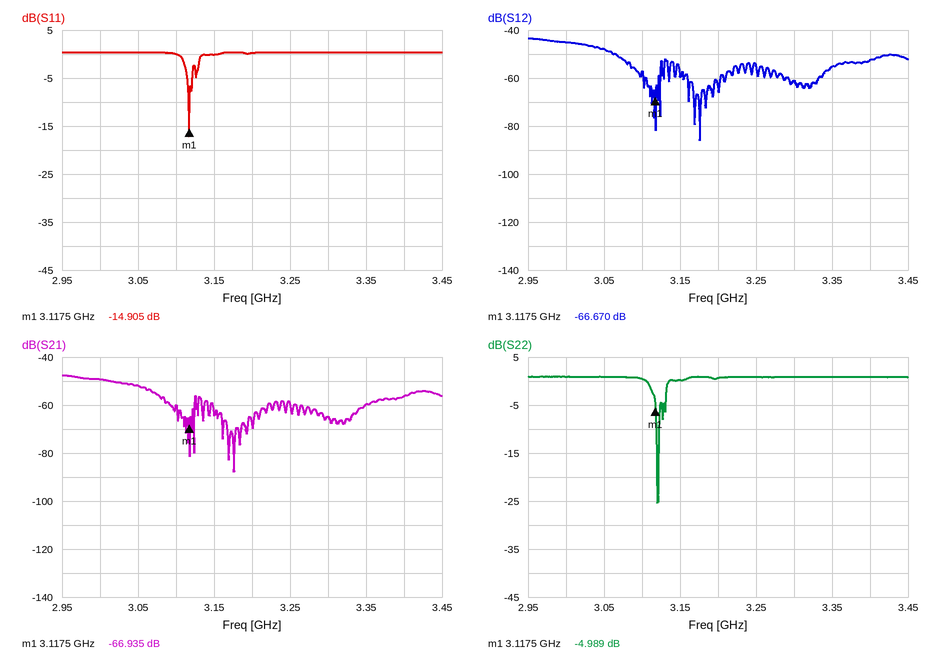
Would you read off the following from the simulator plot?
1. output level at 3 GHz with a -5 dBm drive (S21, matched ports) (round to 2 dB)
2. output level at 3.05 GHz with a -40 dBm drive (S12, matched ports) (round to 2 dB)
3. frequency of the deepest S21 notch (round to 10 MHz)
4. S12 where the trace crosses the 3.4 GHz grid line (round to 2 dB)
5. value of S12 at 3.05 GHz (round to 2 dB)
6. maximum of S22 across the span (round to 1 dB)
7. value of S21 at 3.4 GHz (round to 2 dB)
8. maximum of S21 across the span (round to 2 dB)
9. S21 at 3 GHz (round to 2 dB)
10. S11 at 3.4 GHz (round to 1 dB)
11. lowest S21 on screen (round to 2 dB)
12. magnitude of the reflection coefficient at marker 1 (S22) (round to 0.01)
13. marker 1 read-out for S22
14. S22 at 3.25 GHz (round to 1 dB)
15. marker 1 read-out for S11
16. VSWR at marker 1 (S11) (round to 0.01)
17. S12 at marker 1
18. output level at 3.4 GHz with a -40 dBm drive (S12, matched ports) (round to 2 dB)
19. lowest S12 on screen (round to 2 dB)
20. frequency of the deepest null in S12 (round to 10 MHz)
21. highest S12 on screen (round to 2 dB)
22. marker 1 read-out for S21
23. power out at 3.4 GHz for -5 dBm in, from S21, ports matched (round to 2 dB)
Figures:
-54 dBm
-88 dBm
3.18 GHz
-52 dB
-48 dB
1 dB
-56 dB
-48 dB
-50 dB
0 dB
-88 dB
0.56
-4.989 dB
1 dB
-14.905 dB
1.44
-66.670 dB
-92 dBm
-86 dB
3.18 GHz
-44 dB
-66.935 dB
-62 dBm
